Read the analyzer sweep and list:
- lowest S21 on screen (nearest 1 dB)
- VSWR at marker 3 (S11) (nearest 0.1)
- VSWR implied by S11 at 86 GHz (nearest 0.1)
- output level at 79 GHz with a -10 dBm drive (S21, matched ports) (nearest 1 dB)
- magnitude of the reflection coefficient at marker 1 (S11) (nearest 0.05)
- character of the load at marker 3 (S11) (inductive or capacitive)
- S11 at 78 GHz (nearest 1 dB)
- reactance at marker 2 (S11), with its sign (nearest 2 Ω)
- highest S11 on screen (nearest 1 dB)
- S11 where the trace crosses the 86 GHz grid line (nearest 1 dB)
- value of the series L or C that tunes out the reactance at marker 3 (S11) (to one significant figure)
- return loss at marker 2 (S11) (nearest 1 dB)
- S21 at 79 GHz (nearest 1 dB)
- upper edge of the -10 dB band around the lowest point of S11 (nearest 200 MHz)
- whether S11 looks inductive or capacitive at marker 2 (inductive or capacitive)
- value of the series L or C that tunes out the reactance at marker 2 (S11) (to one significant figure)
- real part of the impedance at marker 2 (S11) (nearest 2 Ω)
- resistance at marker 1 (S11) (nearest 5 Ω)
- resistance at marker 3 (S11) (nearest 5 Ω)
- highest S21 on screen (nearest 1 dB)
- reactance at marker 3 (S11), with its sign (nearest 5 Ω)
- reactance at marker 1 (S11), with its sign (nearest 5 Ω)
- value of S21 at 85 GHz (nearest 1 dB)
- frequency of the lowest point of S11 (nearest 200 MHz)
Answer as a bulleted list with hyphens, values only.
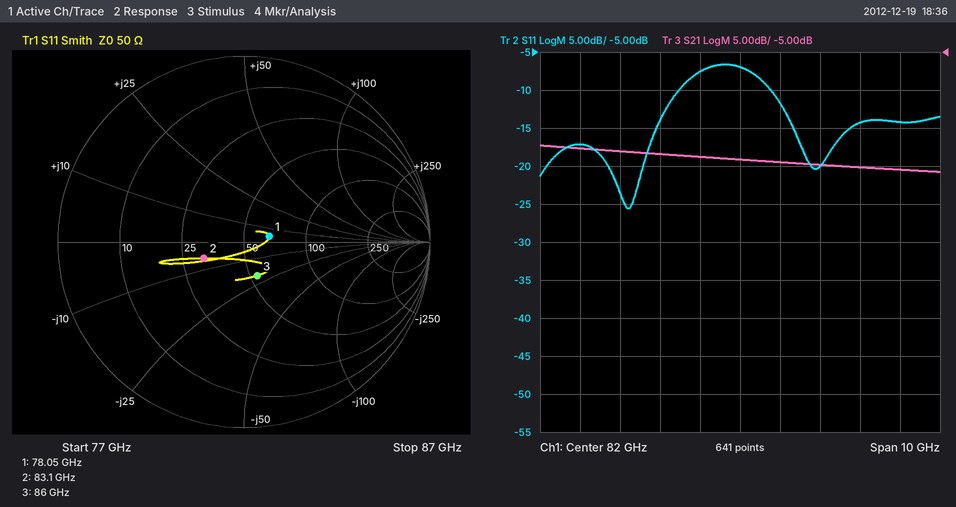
- -21 dB
- 1.5
- 1.5
- -28 dBm
- 0.15
- capacitive
- -17 dB
- -6 Ω
- -7 dB
- -14 dB
- 40 pH
- 13 dB
- -18 dB
- 80.4 GHz
- capacitive
- 10 pH
- 32 Ω
- 65 Ω
- 55 Ω
- -17 dB
- -20 Ω
- +5 Ω
- -20 dB
- 79.2 GHz
